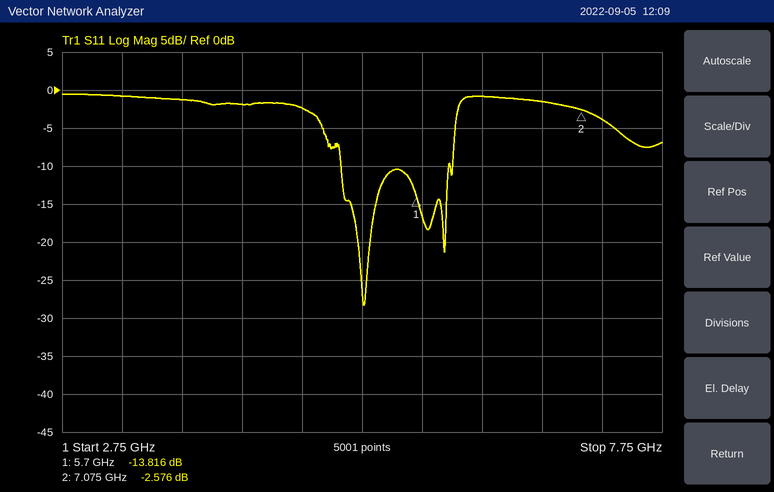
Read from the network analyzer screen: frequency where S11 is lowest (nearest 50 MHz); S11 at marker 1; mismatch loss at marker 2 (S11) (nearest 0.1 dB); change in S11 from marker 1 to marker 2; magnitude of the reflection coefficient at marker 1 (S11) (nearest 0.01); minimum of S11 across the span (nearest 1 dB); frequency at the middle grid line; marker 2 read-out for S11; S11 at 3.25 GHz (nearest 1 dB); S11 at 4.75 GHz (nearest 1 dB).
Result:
5.25 GHz
-13.816 dB
3.5 dB
11.240 dB
0.20
-28 dB
5.25 GHz
-2.576 dB
-1 dB
-2 dB
